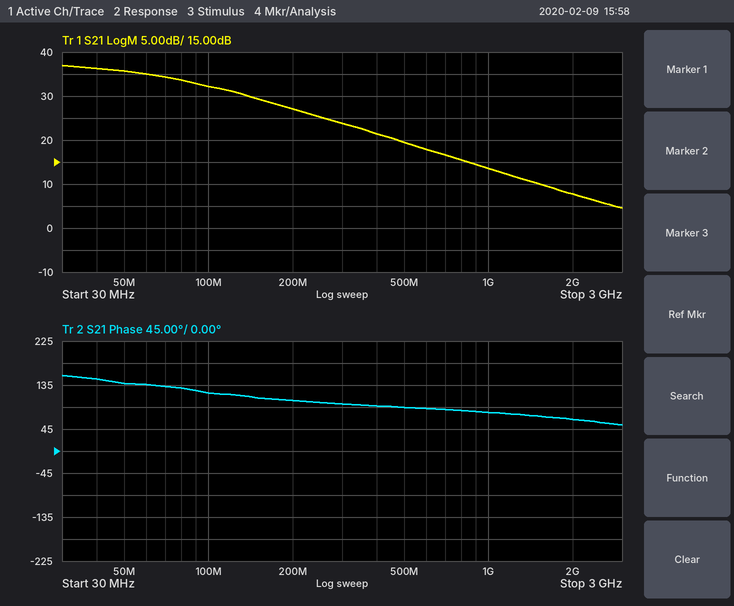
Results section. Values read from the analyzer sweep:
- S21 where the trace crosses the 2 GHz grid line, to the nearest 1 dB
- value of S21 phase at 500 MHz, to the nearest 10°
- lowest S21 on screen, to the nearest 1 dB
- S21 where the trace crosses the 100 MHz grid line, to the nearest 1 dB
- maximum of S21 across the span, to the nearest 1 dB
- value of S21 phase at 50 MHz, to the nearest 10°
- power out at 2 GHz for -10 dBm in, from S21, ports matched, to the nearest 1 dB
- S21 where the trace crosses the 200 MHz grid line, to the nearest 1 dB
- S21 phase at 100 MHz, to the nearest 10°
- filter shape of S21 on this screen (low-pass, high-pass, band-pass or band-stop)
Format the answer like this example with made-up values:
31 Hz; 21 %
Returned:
8 dB; 90°; 5 dB; 32 dB; 37 dB; 140°; -2 dBm; 27 dB; 120°; low-pass
